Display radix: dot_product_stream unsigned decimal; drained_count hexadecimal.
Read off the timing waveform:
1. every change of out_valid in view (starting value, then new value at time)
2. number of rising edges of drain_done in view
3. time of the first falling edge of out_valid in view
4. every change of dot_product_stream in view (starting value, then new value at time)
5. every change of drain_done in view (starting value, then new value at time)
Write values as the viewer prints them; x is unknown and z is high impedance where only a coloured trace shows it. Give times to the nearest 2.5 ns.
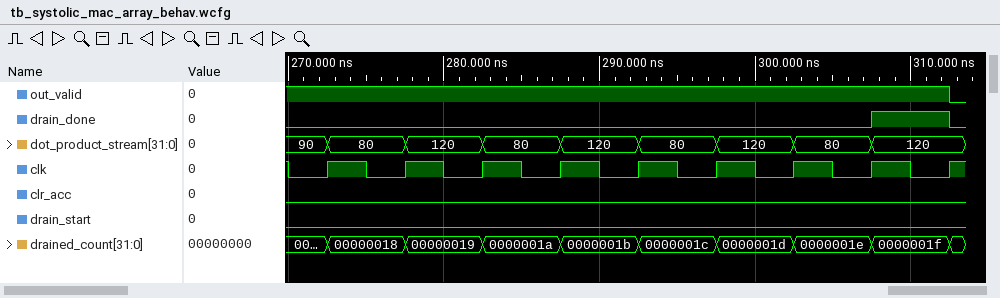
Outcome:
1, 0 at 312.5 ns
1
312.5 ns
90, 80 at 272.5 ns, 120 at 277.5 ns, 80 at 282.5 ns, 120 at 287.5 ns, 80 at 292.5 ns, 120 at 297.5 ns, 80 at 302.5 ns, 120 at 307.5 ns
0, 1 at 307.5 ns, 0 at 312.5 ns
